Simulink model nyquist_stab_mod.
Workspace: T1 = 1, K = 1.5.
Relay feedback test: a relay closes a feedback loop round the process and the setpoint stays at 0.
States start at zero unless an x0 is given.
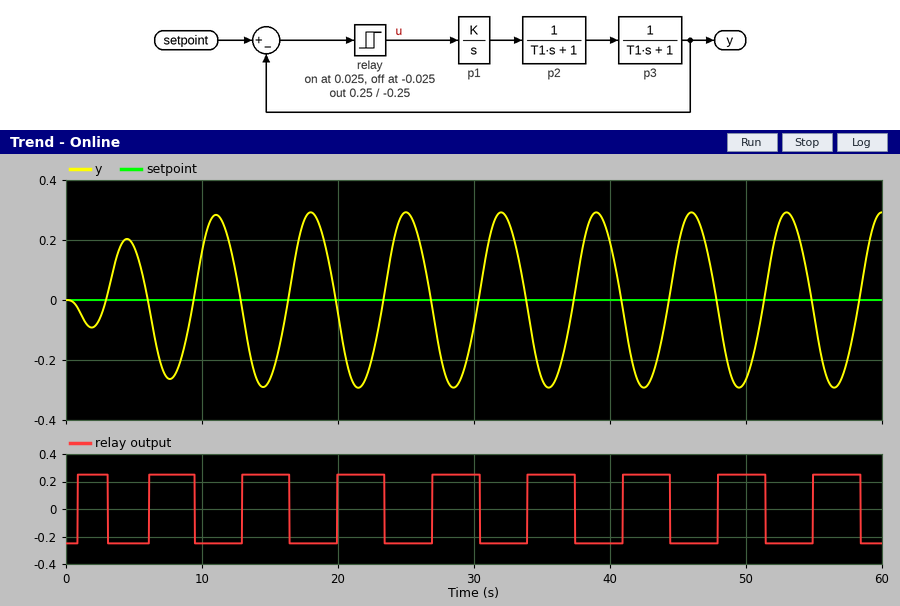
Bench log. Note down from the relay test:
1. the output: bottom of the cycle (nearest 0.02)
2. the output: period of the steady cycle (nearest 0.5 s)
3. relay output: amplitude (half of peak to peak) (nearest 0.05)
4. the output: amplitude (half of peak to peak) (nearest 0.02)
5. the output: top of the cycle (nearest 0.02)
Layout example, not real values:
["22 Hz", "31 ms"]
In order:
["-0.30", "7.0 s", "0.25", "0.30", "0.30"]
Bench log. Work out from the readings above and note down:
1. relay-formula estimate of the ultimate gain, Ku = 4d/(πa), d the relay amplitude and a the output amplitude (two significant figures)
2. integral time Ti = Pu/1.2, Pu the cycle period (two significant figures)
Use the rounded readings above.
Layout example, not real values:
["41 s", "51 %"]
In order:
["1.1", "5.8 s"]
